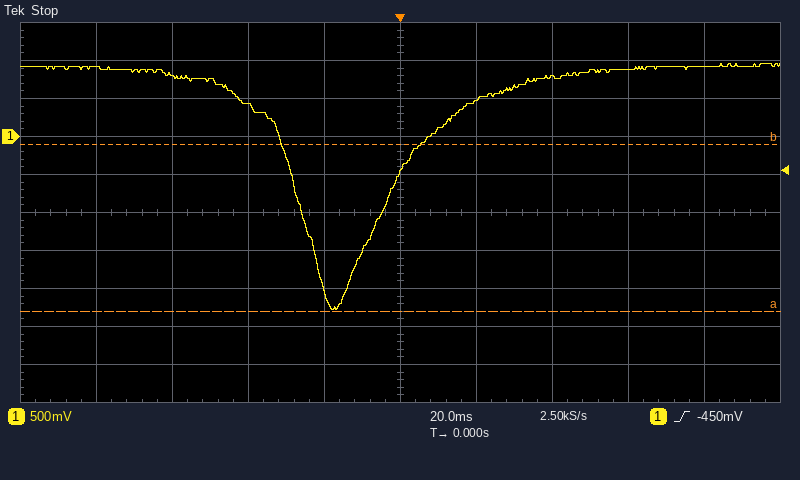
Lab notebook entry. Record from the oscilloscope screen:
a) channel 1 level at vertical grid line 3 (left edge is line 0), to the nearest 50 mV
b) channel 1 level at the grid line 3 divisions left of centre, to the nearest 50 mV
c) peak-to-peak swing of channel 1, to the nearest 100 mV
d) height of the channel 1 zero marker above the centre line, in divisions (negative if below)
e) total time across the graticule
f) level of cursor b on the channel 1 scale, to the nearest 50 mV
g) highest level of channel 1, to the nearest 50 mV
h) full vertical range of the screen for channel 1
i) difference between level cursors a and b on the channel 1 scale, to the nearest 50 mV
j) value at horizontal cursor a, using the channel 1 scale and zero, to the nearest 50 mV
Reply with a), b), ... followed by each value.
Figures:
a) 400 mV
b) 800 mV
c) 3.20 V
d) +2.0 div
e) 200 ms
f) -100 mV
g) 950 mV
h) 5 V
i) 2.20 V
j) -2.30 V
